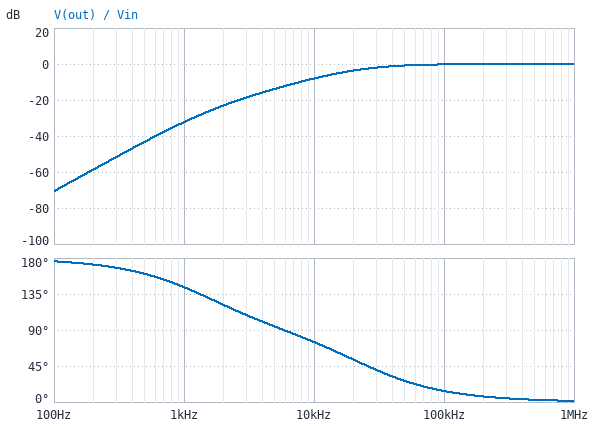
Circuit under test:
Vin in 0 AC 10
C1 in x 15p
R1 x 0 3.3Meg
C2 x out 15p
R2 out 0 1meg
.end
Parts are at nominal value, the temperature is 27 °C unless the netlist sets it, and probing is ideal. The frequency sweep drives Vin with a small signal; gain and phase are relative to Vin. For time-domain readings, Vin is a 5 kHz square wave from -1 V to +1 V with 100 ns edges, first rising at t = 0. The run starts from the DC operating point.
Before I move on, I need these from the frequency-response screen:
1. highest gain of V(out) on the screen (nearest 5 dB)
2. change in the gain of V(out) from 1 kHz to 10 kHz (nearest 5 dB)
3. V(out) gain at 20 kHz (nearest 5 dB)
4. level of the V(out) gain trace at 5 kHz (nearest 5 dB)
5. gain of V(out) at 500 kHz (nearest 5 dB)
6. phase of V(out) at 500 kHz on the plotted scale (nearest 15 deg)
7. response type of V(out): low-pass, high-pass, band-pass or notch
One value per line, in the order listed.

0 dB
25 dB
-5 dB
-15 dB
0 dB
0 deg
high-pass
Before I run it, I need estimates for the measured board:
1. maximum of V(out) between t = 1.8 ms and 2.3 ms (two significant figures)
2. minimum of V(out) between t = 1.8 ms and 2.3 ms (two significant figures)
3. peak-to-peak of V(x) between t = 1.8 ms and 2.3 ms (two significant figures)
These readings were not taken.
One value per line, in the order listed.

2.0 V
-2.0 V
3.5 V
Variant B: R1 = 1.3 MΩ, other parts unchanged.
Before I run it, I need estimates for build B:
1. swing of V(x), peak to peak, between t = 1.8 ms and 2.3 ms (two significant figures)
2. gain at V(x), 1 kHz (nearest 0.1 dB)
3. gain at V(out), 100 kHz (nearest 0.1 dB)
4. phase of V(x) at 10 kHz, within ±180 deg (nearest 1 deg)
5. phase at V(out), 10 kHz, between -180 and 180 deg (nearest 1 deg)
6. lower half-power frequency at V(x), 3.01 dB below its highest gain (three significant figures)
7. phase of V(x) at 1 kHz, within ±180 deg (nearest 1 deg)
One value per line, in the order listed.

3.8 V
-18.6 dB
-0.3 dB
41 deg
87 deg
21.9 kHz
76 deg
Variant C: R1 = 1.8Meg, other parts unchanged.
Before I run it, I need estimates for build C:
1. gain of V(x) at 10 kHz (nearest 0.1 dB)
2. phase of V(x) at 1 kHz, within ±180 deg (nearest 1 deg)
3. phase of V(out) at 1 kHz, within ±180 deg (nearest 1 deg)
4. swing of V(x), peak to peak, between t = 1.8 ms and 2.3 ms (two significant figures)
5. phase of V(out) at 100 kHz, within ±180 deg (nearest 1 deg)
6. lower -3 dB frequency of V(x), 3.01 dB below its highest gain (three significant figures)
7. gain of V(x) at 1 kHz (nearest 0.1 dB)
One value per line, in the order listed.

-5.5 dB
72 deg
156 deg
3.7 V
15 deg
19.9 kHz
-16.0 dB
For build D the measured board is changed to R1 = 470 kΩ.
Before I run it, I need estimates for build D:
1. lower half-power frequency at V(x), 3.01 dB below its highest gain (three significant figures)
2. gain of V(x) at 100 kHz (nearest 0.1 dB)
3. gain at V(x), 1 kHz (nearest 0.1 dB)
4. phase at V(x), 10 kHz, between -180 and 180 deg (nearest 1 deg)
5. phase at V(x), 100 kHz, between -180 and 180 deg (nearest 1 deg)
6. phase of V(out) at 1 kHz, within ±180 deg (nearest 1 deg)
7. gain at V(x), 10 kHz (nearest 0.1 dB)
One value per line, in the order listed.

35.5 kHz
-0.5 dB
-27.1 dB
61 deg
18 deg
170 deg
-10.0 dB
